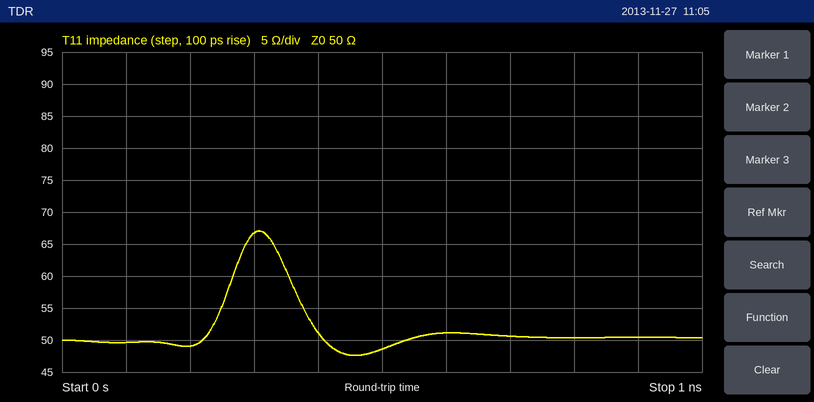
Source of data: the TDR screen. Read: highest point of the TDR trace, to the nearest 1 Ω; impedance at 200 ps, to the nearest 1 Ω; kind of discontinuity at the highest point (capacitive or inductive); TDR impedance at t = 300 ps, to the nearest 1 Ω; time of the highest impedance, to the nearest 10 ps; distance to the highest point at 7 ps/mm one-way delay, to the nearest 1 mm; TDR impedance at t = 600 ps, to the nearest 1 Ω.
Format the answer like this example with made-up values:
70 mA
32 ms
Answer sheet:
67 Ω
49 Ω
inductive
67 Ω
310 ps
22 mm
51 Ω
